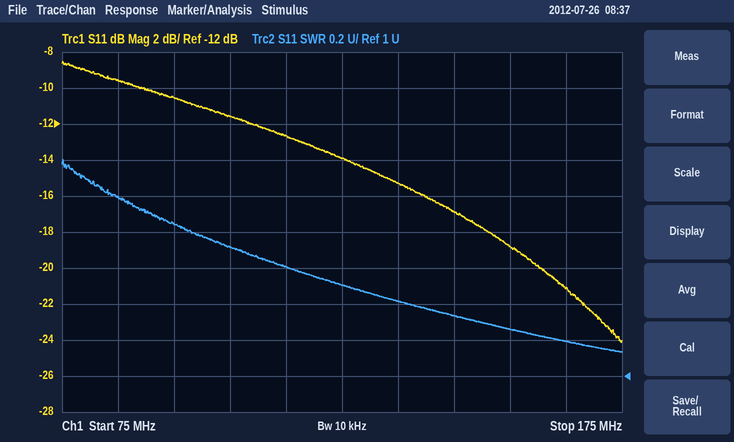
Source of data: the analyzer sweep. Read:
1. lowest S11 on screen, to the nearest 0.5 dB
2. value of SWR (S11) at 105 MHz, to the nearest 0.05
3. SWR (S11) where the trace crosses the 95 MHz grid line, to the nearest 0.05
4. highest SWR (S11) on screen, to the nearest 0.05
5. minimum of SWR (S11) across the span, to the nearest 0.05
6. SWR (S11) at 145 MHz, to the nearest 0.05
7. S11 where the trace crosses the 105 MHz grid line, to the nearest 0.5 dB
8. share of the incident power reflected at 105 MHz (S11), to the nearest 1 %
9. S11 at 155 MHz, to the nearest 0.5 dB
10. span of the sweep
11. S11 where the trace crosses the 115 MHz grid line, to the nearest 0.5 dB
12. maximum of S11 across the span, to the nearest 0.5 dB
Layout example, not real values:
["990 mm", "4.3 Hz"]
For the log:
["-24.0 dB", "1.70", "1.85", "2.20", "1.15", "1.35", "-11.5 dB", "7 %", "-19.0 dB", "100 MHz", "-12.5 dB", "-8.5 dB"]
